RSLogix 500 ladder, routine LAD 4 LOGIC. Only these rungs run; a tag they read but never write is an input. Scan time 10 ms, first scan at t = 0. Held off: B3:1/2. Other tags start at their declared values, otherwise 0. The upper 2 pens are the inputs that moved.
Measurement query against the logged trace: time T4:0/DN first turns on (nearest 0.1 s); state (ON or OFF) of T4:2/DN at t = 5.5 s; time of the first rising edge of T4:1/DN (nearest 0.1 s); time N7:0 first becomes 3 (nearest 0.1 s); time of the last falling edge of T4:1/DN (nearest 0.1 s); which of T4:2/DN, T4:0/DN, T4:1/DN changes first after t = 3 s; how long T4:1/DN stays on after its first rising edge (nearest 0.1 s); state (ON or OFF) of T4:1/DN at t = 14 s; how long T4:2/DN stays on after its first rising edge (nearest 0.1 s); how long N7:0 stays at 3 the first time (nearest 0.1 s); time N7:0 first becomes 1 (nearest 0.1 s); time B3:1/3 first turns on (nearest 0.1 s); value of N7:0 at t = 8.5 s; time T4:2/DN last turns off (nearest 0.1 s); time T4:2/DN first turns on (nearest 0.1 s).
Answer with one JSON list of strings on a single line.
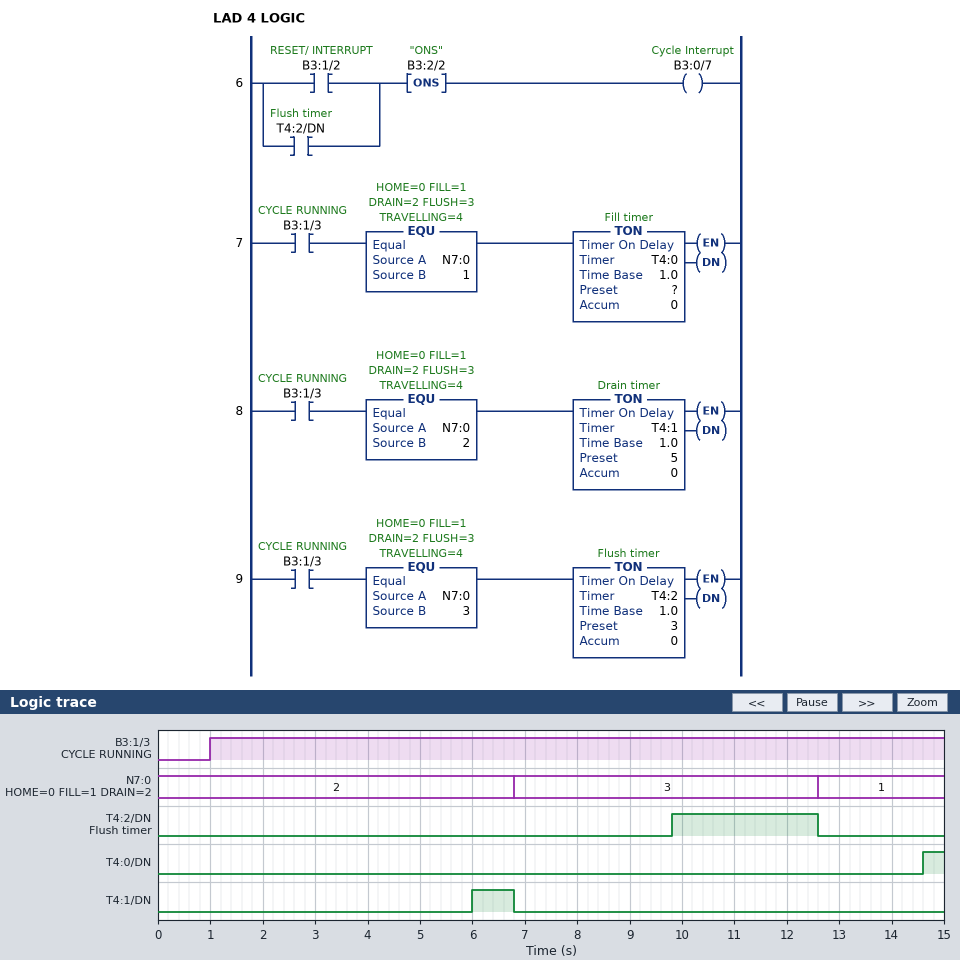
["14.6 s", "OFF", "6.0 s", "6.8 s", "6.8 s", "T4:1/DN", "0.8 s", "OFF", "2.8 s", "5.8 s", "12.6 s", "1.0 s", "3", "12.6 s", "9.8 s"]
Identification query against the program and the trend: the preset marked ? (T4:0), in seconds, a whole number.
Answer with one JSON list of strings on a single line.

["2 s"]
